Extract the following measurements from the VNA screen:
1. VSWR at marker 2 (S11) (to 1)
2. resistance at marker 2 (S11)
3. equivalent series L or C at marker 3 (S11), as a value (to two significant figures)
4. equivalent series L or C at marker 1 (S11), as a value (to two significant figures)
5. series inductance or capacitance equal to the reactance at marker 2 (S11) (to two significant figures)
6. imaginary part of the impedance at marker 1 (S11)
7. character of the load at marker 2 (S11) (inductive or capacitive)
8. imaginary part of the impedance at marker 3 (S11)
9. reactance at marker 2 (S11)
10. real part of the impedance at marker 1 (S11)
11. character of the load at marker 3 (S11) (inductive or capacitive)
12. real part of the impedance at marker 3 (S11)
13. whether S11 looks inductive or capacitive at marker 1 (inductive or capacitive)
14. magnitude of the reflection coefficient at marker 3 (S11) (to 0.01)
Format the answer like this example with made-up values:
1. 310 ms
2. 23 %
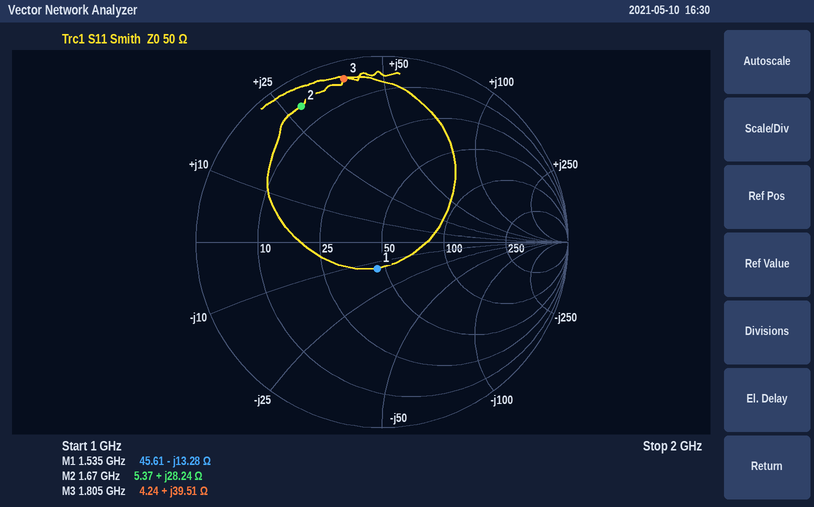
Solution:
1. 12
2. 5.37 Ω
3. 3.5 nH
4. 7.8 pF
5. 2.7 nH
6. -13.28 Ω
7. inductive
8. +39.51 Ω
9. +28.24 Ω
10. 45.61 Ω
11. inductive
12. 4.24 Ω
13. capacitive
14. 0.90
